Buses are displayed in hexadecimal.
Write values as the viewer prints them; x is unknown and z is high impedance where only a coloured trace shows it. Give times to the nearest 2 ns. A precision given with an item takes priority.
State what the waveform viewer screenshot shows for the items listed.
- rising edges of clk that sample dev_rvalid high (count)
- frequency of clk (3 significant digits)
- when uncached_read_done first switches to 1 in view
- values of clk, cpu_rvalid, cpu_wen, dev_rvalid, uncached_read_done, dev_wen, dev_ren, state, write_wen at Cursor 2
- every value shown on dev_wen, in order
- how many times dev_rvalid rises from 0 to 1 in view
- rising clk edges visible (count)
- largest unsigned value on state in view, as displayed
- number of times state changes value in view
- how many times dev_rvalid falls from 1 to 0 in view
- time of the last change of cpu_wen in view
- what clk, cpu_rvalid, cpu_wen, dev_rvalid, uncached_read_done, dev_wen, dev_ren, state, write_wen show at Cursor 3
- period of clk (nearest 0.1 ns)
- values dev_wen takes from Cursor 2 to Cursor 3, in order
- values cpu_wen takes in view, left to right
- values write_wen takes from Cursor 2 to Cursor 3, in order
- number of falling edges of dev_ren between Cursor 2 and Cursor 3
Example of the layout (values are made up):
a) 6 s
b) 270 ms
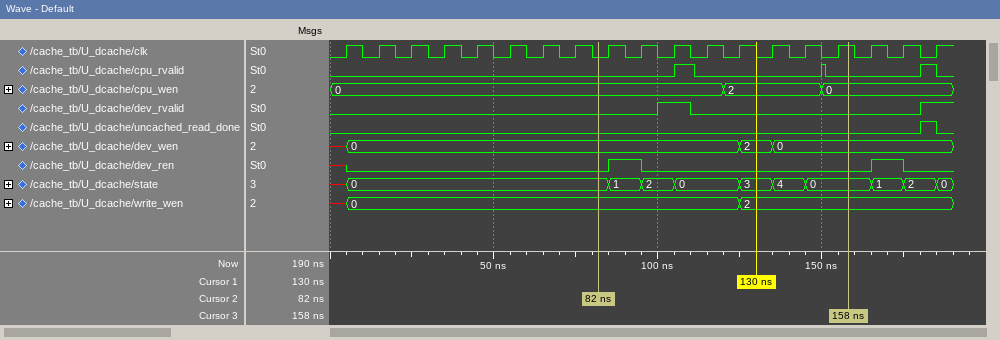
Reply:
a) 2
b) 100 MHz
c) 180 ns
d) clk=0, cpu_rvalid=0, cpu_wen=0, dev_rvalid=0, uncached_read_done=0, dev_wen=0, dev_ren=0, state=0, write_wen=0
e) x, 0, 2, 0
f) 2
g) 19
h) 4
i) 10
j) 1
k) 150 ns
l) clk=1, cpu_rvalid=0, cpu_wen=0, dev_rvalid=0, uncached_read_done=0, dev_wen=0, dev_ren=0, state=0, write_wen=2
m) 10 ns
n) 0, 2, 0
o) 0, 2, 0
p) 0, 2
q) 1
